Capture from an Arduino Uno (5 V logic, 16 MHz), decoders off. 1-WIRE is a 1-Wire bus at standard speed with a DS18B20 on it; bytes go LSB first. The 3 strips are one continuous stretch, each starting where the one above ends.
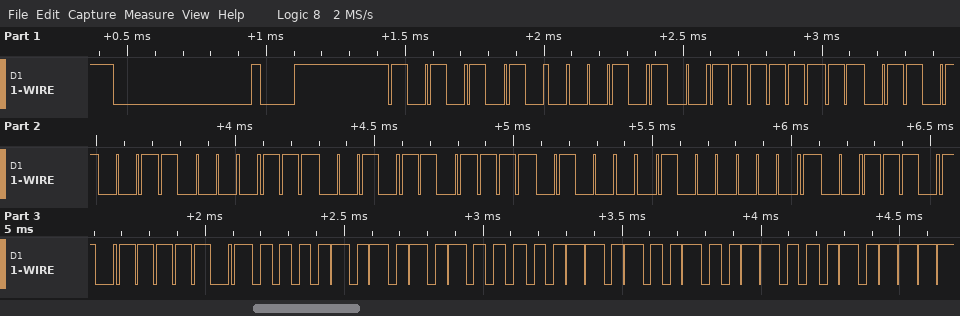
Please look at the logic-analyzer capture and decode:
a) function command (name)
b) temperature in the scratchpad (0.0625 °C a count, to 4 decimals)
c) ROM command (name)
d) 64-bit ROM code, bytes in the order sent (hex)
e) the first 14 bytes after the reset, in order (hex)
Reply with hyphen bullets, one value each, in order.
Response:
- Read Scratchpad
- 85.0000 °C
- Match ROM
- 28 FF 96 E1 B4 17 02 B9
- 55 28 FF 96 E1 B4 17 02 B9 BE 50 05 4B 46
